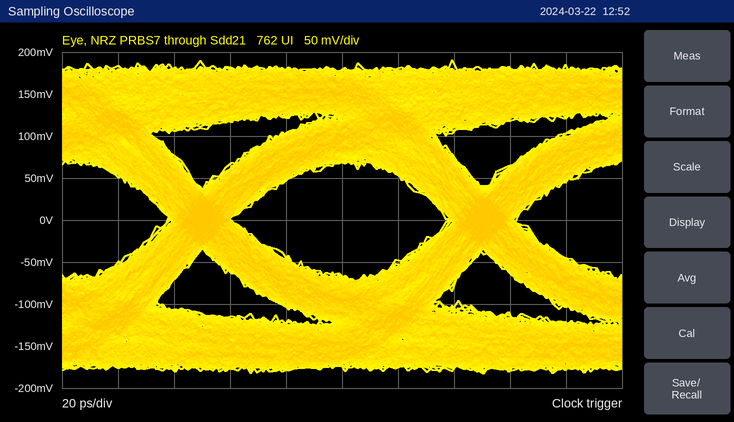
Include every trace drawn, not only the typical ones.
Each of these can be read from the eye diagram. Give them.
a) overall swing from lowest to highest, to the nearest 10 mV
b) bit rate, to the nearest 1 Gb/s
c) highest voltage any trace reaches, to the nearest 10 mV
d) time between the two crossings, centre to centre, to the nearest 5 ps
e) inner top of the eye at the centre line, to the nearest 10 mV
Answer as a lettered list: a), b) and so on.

a) 370 mV
b) 10 Gb/s
c) 190 mV
d) 100 ps
e) 70 mV
